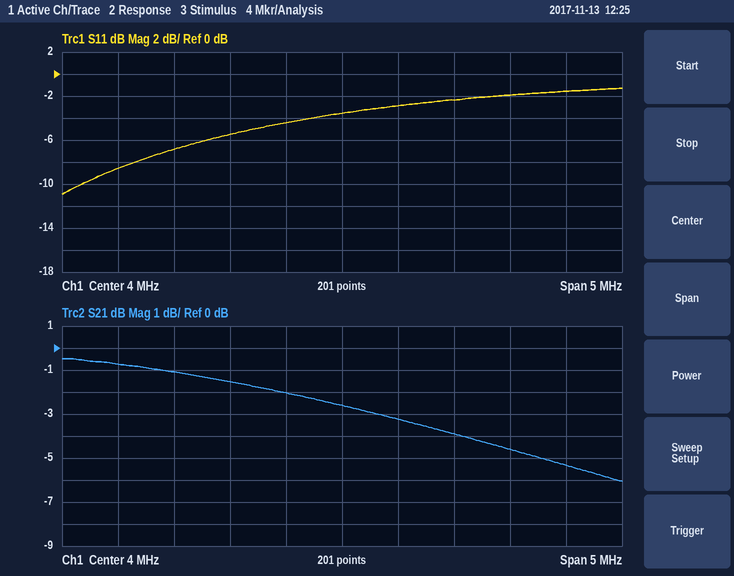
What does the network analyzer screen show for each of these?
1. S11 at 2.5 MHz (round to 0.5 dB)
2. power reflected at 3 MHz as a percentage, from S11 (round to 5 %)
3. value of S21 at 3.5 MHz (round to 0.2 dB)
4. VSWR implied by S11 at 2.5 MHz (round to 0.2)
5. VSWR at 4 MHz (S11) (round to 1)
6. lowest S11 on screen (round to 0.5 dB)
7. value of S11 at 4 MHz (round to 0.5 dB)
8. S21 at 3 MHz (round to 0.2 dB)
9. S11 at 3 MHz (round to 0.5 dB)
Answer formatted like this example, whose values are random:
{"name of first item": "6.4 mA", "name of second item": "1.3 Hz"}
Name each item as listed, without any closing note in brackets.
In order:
{"S11 at 2.5 MHz": "-7.0 dB", "power reflected at 3 MHz as a percentage, from S11": "30 %", "value of S21 at 3.5 MHz": "-2.0 dB", "VSWR implied by S11 at 2.5 MHz": "2.6", "VSWR at 4 MHz (S11)": "5", "lowest S11 on screen": "-11.0 dB", "value of S11 at 4 MHz": "-3.5 dB", "S21 at 3 MHz": "-1.6 dB", "S11 at 3 MHz": "-5.5 dB"}
